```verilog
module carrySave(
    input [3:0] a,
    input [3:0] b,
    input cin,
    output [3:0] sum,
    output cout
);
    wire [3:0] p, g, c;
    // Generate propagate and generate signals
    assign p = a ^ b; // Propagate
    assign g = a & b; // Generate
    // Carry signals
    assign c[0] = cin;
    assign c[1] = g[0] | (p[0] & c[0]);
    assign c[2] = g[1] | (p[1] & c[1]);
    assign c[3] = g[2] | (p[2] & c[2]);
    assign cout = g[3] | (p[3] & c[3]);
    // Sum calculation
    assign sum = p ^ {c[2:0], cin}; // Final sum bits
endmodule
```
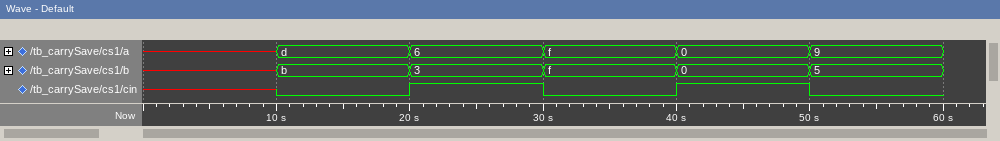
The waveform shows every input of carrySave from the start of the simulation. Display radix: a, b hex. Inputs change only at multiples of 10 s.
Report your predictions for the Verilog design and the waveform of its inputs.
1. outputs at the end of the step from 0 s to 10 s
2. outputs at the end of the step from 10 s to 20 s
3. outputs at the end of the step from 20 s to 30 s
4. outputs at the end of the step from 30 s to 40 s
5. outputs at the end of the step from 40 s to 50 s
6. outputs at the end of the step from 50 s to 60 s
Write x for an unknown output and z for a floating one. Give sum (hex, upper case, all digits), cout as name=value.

sum=x, cout=x
sum=A, cout=1
sum=A, cout=0
sum=C, cout=1
sum=3, cout=0
sum=8, cout=0
